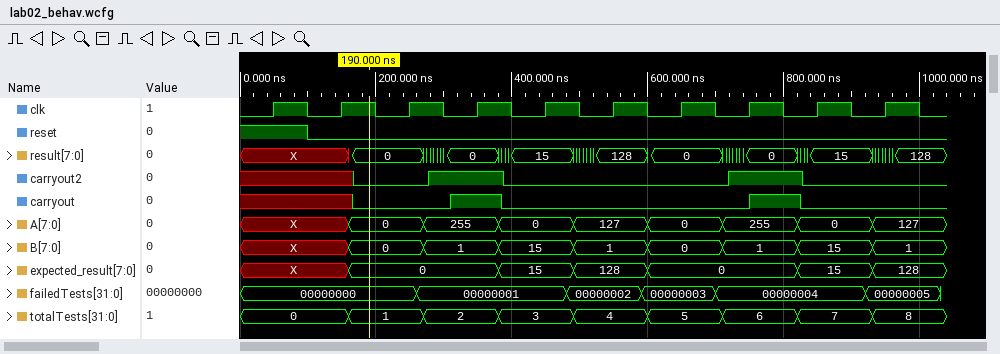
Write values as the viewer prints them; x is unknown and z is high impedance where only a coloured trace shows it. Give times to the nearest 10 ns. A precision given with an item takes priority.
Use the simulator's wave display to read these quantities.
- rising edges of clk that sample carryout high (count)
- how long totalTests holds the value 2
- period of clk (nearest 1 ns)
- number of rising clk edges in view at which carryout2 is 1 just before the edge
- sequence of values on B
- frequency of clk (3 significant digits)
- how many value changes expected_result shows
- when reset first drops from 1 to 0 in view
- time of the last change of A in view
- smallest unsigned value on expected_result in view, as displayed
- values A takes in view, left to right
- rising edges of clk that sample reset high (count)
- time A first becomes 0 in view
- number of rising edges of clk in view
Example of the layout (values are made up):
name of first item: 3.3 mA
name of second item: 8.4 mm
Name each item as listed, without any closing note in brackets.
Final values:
rising edges of clk that sample carryout high: 1
how long totalTests holds the value 2: 110 ns
period of clk: 100 ns
number of rising clk edges in view at which carryout2 is 1 just before the edge: 2
sequence of values on B: X, 0, 1, 15, 1, 0, 1, 15, 1
frequency of clk: 10.0 MHz
how many value changes expected_result shows: 6
when reset first drops from 1 to 0 in view: 100 ns
time of the last change of A in view: 930 ns
smallest unsigned value on expected_result in view, as displayed: 0
values A takes in view, left to right: X, 0, 255, 0, 127, 0, 255, 0, 127
rising edges of clk that sample reset high: 1
time A first becomes 0 in view: 160 ns
number of rising edges of clk in view: 10
